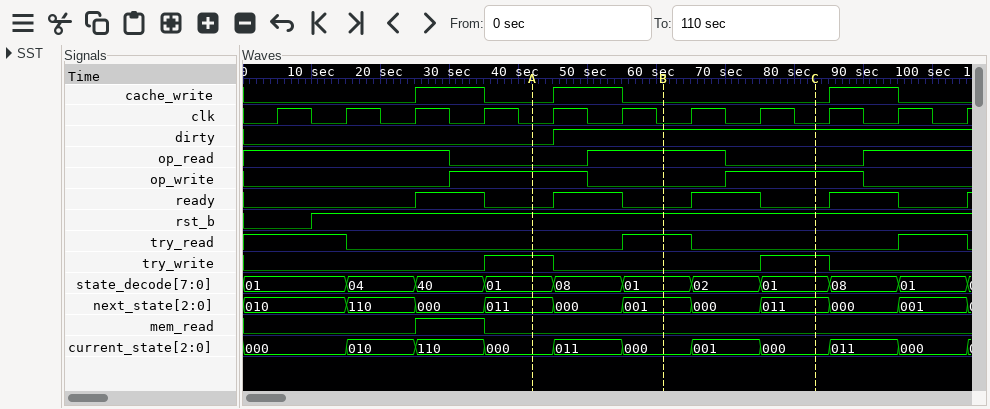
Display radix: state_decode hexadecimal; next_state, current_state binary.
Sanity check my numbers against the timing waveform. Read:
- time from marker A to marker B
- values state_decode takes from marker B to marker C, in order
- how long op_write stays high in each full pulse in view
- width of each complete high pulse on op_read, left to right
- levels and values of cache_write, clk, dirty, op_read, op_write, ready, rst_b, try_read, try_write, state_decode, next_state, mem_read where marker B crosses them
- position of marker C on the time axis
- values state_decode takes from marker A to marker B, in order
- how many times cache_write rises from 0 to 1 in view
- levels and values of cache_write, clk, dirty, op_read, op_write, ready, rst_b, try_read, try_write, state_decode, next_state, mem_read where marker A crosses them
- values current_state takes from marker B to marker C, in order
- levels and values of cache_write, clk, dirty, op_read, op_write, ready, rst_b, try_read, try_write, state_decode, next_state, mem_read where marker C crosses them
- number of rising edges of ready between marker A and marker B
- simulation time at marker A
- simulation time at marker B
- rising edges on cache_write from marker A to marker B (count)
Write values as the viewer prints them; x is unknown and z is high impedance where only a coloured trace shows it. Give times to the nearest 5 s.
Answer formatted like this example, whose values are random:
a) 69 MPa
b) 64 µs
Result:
a) 20 s
b) 01, 02, 01
c) 20 s, 20 s
d) 20 s
e) cache_write=0, clk=0, dirty=1, op_read=1, op_write=0, ready=0, rst_b=1, try_read=1, try_write=0, state_decode=01, next_state=001, mem_read=0
f) 85 s
g) 01, 08, 01
h) 3
i) cache_write=0, clk=0, dirty=0, op_read=0, op_write=1, ready=0, rst_b=1, try_read=0, try_write=1, state_decode=01, next_state=011, mem_read=0
j) 000, 001, 000
k) cache_write=0, clk=0, dirty=1, op_read=0, op_write=1, ready=0, rst_b=1, try_read=0, try_write=1, state_decode=01, next_state=011, mem_read=0
l) 1
m) 40 s
n) 60 s
o) 1
